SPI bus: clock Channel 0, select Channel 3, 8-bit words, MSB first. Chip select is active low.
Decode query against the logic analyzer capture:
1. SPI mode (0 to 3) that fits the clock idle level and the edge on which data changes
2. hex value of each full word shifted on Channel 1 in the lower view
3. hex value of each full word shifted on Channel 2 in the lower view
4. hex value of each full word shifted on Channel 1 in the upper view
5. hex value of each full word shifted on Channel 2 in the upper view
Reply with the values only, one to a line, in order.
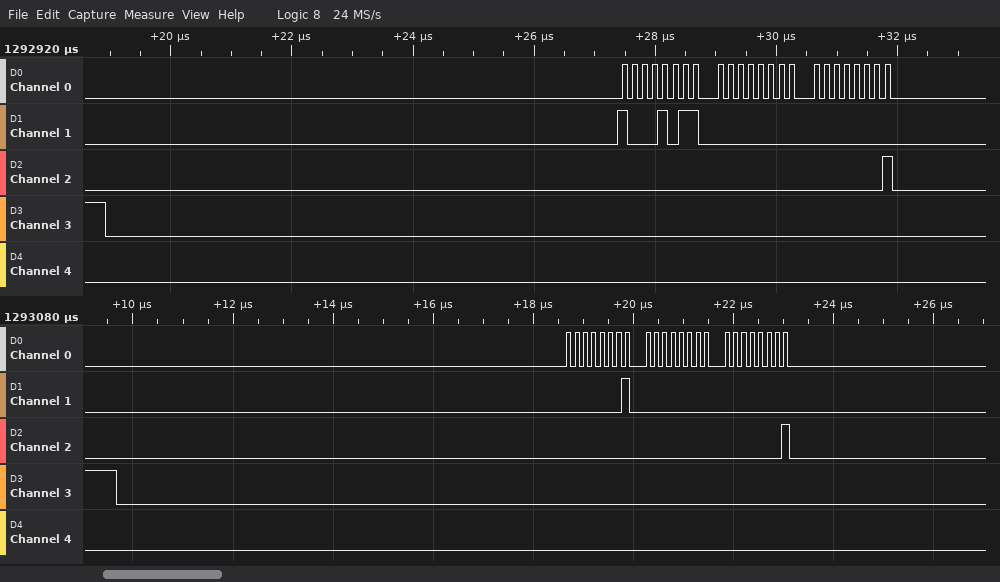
0
01, 00, 00
00, 00, 01
8B, 00, 00
00, 00, 01
